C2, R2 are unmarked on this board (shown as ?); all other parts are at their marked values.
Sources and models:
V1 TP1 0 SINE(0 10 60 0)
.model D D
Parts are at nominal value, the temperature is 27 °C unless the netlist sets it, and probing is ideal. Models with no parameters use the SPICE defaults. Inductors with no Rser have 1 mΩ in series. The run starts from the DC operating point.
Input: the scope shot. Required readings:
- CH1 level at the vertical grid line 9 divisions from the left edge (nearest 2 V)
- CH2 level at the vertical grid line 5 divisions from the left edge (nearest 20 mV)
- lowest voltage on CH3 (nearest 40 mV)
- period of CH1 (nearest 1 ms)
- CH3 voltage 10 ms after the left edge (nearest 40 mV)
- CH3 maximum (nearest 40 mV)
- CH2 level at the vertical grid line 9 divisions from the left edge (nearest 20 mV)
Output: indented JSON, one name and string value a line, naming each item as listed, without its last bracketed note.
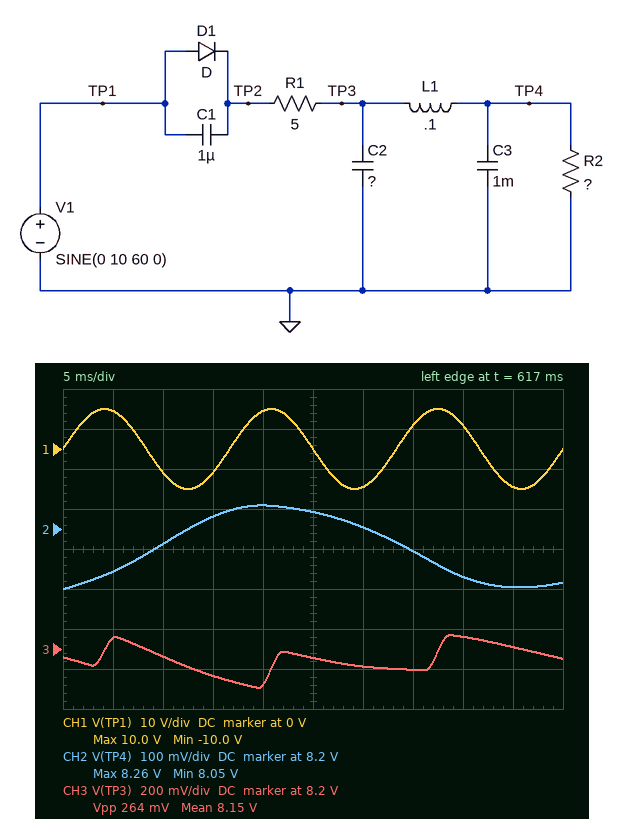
{
  "CH1 level at the vertical grid line 9 divisions from the left edge": "-10 V",
  "CH2 level at the vertical grid line 5 divisions from the left edge": "8.24 V",
  "lowest voltage on CH3": "8.00 V",
  "period of CH1": "17 ms",
  "CH3 voltage 10 ms after the left edge": "8.16 V",
  "CH3 maximum": "8.28 V",
  "CH2 level at the vertical grid line 9 divisions from the left edge": "8.06 V"
}
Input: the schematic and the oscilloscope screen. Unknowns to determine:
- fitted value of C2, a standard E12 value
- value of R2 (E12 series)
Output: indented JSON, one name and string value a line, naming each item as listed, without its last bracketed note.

{
  "fitted value of C2, a standard E12 value": "1.8 mF",
  "value of R2": "390 Ω"
}
